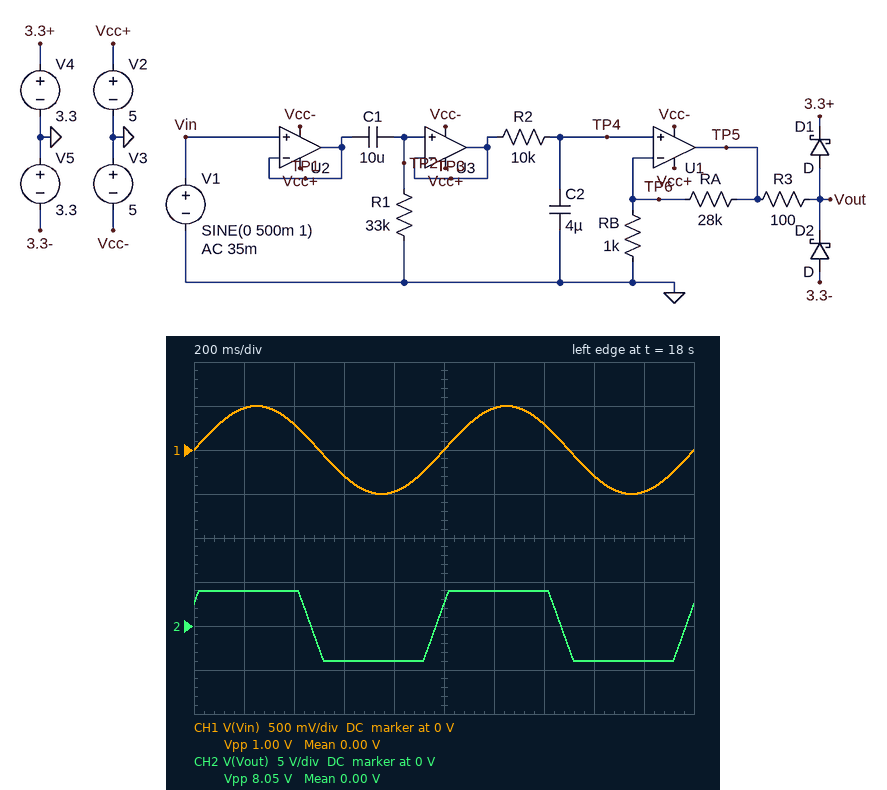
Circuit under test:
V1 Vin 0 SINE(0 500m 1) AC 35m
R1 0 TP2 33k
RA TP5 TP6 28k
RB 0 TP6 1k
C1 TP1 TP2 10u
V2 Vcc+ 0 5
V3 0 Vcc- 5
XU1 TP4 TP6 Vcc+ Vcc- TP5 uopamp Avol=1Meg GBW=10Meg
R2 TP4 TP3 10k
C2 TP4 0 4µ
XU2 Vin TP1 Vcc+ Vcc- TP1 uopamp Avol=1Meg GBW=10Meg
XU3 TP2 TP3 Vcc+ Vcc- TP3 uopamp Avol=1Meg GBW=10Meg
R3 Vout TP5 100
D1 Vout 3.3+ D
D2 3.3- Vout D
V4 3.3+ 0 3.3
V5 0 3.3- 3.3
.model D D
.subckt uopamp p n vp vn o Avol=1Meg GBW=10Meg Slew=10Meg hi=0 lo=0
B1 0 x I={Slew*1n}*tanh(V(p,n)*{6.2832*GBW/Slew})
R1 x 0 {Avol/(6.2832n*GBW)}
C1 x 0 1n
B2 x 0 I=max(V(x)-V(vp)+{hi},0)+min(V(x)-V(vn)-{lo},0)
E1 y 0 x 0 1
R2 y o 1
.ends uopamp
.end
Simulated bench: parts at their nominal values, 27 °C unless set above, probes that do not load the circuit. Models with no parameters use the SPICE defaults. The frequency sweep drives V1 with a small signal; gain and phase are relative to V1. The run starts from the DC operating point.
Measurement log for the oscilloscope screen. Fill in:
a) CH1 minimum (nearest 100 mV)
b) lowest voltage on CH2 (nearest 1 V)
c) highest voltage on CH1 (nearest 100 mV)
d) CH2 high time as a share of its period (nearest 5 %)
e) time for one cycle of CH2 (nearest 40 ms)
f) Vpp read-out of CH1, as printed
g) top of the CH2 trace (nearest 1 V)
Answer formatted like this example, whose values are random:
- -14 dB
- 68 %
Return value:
- -500 mV
- -4 V
- 500 mV
- 50 %
- 1.00 s
- 1.00 V
- 4 V
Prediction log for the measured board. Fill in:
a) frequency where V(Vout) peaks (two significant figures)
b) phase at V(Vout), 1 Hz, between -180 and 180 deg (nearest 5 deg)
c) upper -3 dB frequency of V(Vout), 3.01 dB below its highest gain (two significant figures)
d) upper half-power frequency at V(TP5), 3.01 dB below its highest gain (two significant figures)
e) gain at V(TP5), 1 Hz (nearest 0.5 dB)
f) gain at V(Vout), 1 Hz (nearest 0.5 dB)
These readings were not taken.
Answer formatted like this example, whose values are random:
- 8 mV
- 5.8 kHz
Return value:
- 1.4 Hz
- 10 deg
- 4.9 Hz
- 4.9 Hz
- 28.0 dB
- 28.0 dB
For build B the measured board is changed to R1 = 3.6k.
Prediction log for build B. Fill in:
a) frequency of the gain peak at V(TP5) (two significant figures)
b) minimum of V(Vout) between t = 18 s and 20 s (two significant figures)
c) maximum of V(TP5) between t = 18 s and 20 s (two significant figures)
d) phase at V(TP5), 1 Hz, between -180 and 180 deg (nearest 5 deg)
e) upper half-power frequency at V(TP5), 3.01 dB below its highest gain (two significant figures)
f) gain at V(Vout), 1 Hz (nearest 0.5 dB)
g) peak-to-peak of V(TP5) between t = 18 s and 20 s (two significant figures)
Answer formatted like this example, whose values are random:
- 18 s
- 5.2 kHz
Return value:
- 4.2 Hz
- -3.1 V
- 3.1 V
- 65 deg
- 10 Hz
- 16.0 dB
- 6.2 V
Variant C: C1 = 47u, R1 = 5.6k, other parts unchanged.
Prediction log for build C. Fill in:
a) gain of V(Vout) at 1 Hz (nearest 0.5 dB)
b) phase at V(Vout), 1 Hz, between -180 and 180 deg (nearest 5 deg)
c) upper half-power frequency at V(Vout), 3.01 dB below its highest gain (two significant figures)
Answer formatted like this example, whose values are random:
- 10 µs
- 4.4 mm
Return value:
- 27.5 dB
- 15 deg
- 5.1 Hz
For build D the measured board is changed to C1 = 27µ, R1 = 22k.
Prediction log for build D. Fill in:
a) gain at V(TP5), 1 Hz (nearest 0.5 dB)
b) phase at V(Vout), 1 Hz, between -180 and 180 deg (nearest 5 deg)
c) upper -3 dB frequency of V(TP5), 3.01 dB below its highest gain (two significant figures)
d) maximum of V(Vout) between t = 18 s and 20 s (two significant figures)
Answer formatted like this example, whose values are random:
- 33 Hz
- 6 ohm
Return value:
- 28.5 dB
- 0 deg
- 4.5 Hz
- 4.0 V
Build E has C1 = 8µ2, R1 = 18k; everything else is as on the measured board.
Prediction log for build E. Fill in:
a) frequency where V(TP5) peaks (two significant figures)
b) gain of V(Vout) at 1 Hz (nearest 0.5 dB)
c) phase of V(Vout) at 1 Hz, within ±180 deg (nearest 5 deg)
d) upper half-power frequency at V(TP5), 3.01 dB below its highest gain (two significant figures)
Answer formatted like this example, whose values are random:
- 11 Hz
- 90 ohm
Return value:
- 2.1 Hz
- 25.5 dB
- 35 deg
- 5.8 Hz
